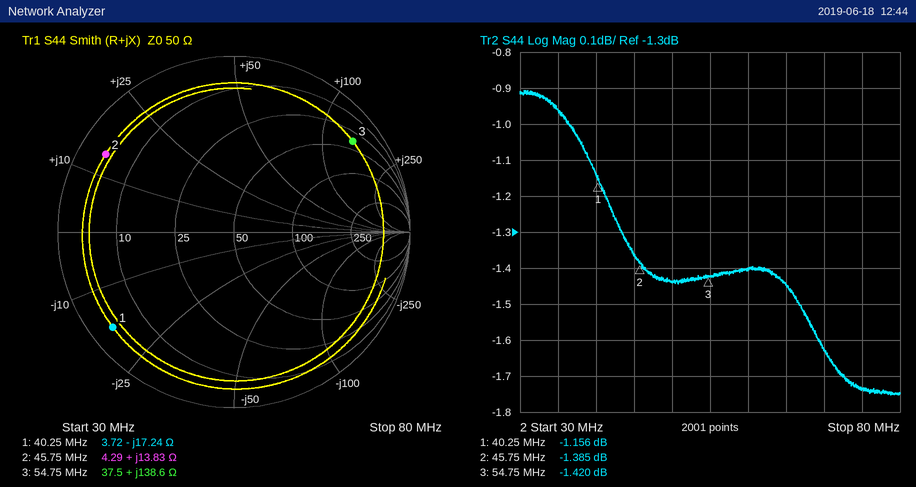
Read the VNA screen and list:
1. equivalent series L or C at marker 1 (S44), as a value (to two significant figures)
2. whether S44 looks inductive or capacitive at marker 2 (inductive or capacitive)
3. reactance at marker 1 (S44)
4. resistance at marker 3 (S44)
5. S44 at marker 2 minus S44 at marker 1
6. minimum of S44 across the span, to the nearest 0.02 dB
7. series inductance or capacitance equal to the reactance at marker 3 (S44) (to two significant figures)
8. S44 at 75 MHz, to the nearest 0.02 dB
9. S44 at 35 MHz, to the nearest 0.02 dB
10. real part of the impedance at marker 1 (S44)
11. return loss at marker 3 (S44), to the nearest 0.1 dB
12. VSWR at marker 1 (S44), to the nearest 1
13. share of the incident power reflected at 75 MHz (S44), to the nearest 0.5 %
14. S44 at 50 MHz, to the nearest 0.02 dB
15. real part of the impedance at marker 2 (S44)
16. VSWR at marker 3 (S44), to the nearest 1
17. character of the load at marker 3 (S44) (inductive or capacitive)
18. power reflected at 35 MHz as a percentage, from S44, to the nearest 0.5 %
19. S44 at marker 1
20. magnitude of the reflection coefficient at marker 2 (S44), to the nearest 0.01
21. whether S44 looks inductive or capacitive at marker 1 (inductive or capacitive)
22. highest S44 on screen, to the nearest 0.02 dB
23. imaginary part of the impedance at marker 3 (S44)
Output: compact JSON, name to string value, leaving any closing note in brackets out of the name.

{"equivalent series L or C at marker 1 (S44), as a value": "230 pF", "whether S44 looks inductive or capacitive at marker 2": "inductive", "reactance at marker 1": "-17.24 Ω", "resistance at marker 3": "37.5 Ω", "S44 at marker 2 minus S44 at marker 1": "-0.229 dB", "minimum of S44 across the span, to the nearest 0.02 dB": "-1.76 dB", "series inductance or capacitance equal to the reactance at marker 3 (S44)": "400 nH", "S44 at 75 MHz, to the nearest 0.02 dB": "-1.74 dB", "S44 at 35 MHz, to the nearest 0.02 dB": "-0.96 dB", "real part of the impedance at marker 1": "3.72 Ω", "return loss at marker 3 (S44), to the nearest 0.1 dB": "1.4 dB", "VSWR at marker 1 (S44), to the nearest 1": "15", "share of the incident power reflected at 75 MHz (S44), to the nearest 0.5 %": "67.0 %", "S44 at 50 MHz, to the nearest 0.02 dB": "-1.44 dB", "real part of the impedance at marker 2": "4.29 Ω", "VSWR at marker 3 (S44), to the nearest 1": "12", "character of the load at marker 3 (S44)": "inductive", "power reflected at 35 MHz as a percentage, from S44, to the nearest 0.5 %": "80.0 %", "S44 at marker 1": "-1.156 dB", "magnitude of the reflection coefficient at marker 2 (S44), to the nearest 0.01": "0.85", "whether S44 looks inductive or capacitive at marker 1": "capacitive", "highest S44 on screen, to the nearest 0.02 dB": "-0.90 dB", "imaginary part of the impedance at marker 3": "+138.6 Ω"}
